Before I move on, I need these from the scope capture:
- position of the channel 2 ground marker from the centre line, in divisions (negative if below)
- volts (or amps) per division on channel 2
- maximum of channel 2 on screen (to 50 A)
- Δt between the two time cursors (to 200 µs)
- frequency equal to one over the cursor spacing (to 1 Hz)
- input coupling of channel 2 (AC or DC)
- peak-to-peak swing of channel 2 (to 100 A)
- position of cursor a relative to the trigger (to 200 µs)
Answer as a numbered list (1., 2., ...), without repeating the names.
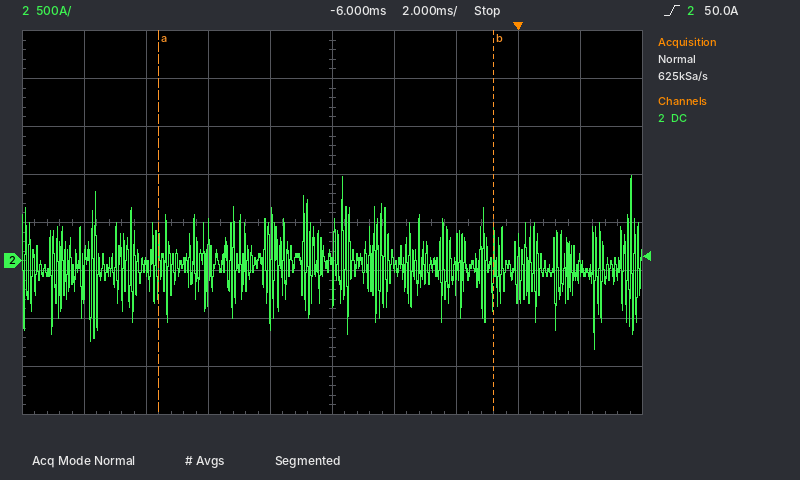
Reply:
1. -0.8 div
2. 500 A
3. 900 A
4. 10.8 ms
5. 93 Hz
6. DC
7. 1.80 kA
8. -11.6 ms
